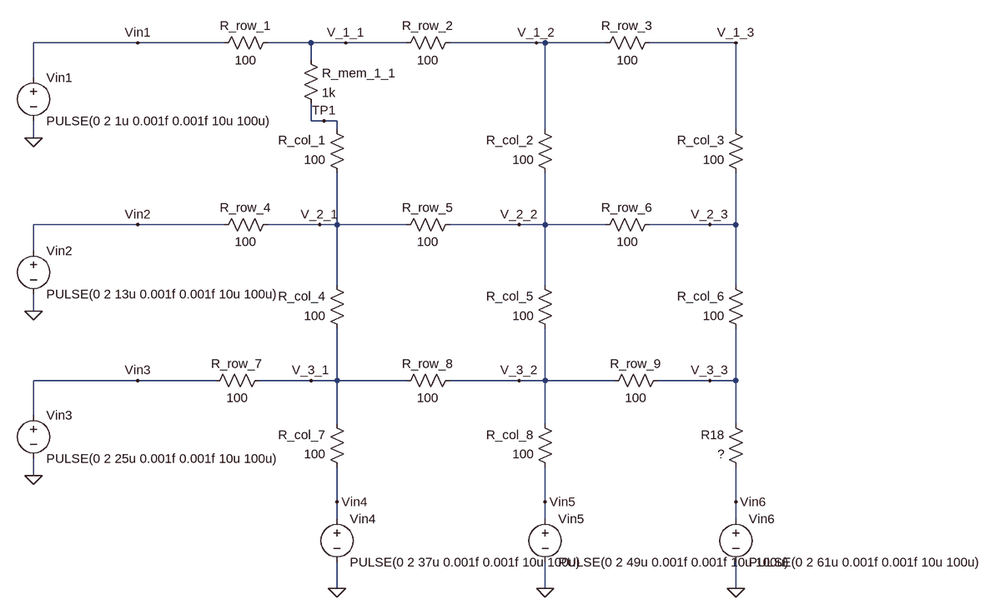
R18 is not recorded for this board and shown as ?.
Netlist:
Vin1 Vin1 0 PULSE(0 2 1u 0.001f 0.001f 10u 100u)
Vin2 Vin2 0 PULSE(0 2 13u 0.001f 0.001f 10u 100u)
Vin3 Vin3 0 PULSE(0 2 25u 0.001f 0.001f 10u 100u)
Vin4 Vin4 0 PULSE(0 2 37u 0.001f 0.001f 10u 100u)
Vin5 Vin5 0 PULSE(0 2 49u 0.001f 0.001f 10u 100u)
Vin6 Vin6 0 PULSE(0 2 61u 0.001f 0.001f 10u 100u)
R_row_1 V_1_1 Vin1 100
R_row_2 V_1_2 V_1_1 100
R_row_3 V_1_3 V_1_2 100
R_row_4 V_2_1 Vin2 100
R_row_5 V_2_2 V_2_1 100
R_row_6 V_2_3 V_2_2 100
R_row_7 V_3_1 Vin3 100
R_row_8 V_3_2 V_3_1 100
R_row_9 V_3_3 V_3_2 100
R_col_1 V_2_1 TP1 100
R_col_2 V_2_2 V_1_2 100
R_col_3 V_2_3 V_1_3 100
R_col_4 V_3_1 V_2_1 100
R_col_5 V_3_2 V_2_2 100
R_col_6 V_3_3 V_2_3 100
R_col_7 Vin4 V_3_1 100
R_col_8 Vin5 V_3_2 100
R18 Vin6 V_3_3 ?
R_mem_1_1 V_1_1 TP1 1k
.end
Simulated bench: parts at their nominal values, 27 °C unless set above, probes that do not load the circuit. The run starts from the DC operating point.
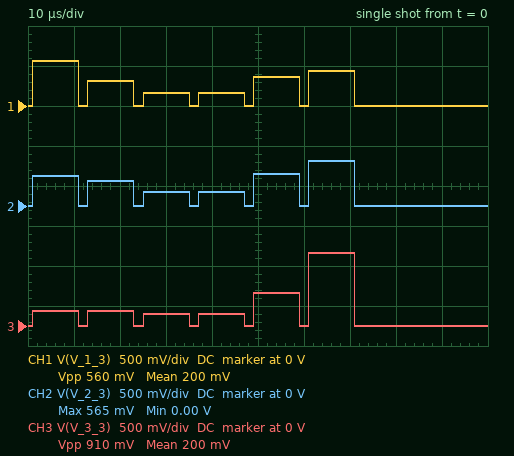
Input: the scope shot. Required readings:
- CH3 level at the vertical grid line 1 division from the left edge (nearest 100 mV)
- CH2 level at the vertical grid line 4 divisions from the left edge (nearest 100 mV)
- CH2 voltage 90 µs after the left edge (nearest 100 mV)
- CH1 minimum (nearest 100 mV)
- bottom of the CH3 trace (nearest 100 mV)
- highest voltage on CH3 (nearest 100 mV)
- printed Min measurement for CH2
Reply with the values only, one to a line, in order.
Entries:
200 mV
200 mV
0 V
0 V
0 V
900 mV
0.00 V
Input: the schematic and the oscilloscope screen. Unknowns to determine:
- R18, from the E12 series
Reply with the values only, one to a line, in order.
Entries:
120 Ω
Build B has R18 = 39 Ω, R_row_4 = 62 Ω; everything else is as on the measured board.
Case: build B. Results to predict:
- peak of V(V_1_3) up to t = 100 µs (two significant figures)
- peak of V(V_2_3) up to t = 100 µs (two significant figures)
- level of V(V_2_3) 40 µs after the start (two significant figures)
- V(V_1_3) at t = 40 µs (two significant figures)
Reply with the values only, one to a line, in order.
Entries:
680 mV
880 mV
120 mV
110 mV
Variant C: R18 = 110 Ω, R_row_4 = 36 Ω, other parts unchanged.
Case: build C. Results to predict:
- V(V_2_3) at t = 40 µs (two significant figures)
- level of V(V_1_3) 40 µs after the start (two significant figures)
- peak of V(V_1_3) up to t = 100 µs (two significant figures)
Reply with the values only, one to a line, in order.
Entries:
130 mV
120 mV
530 mV
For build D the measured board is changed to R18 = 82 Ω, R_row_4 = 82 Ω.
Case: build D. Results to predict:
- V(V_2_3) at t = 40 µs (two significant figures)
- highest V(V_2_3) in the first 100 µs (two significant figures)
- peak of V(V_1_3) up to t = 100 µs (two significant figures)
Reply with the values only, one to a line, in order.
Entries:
150 mV
680 mV
540 mV
